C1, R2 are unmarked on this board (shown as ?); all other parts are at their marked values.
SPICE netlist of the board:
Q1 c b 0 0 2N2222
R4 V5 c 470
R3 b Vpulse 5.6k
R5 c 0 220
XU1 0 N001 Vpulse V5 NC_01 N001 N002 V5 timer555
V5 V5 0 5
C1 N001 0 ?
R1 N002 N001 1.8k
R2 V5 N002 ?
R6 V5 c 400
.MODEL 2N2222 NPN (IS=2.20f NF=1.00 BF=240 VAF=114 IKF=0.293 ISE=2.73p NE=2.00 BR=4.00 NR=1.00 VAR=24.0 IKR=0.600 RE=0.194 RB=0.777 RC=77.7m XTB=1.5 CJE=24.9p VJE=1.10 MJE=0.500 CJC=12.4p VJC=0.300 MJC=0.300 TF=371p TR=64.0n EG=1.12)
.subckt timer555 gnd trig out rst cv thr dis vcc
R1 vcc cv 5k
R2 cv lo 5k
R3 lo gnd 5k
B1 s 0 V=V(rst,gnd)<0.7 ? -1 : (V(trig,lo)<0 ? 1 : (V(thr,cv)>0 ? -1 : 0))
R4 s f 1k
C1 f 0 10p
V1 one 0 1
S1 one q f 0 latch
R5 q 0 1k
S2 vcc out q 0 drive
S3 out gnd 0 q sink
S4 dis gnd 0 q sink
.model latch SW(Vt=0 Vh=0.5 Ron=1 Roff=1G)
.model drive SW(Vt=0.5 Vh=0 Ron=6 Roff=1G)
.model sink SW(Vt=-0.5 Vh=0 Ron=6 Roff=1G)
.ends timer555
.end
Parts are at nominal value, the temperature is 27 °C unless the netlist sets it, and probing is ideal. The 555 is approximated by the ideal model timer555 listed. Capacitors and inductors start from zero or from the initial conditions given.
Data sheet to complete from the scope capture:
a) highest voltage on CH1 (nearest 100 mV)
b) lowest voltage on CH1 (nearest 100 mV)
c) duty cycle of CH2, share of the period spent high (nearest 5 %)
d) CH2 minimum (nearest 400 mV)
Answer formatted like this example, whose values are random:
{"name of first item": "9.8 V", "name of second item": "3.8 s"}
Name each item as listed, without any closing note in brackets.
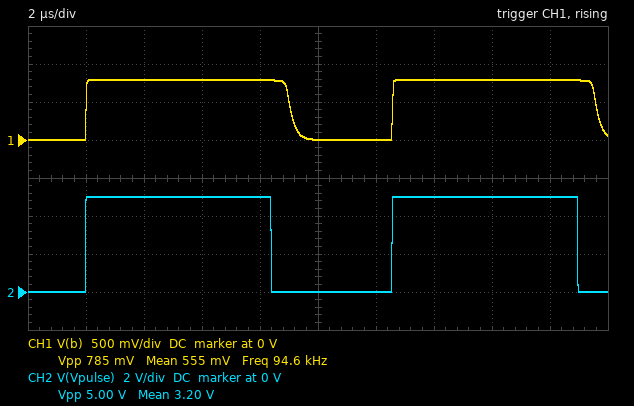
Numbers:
{"highest voltage on CH1": "800 mV", "lowest voltage on CH1": "0 V", "duty cycle of CH2, share of the period spent high": "60 %", "CH2 minimum": "0 V"}
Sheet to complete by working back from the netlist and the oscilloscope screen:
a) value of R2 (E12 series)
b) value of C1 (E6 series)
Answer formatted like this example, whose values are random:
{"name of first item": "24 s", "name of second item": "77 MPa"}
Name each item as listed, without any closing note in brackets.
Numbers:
{"value of R2": "1 kΩ", "value of C1": "3.3 nF"}
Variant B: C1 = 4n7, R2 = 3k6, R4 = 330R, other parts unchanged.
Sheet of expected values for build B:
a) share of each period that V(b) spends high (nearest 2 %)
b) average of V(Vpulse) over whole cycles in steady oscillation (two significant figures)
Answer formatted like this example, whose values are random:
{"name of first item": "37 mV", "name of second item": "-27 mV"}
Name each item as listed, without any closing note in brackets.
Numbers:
{"share of each period that V(b) spends high": "78 %", "average of V(Vpulse) over whole cycles in steady oscillation": "3.7 V"}
